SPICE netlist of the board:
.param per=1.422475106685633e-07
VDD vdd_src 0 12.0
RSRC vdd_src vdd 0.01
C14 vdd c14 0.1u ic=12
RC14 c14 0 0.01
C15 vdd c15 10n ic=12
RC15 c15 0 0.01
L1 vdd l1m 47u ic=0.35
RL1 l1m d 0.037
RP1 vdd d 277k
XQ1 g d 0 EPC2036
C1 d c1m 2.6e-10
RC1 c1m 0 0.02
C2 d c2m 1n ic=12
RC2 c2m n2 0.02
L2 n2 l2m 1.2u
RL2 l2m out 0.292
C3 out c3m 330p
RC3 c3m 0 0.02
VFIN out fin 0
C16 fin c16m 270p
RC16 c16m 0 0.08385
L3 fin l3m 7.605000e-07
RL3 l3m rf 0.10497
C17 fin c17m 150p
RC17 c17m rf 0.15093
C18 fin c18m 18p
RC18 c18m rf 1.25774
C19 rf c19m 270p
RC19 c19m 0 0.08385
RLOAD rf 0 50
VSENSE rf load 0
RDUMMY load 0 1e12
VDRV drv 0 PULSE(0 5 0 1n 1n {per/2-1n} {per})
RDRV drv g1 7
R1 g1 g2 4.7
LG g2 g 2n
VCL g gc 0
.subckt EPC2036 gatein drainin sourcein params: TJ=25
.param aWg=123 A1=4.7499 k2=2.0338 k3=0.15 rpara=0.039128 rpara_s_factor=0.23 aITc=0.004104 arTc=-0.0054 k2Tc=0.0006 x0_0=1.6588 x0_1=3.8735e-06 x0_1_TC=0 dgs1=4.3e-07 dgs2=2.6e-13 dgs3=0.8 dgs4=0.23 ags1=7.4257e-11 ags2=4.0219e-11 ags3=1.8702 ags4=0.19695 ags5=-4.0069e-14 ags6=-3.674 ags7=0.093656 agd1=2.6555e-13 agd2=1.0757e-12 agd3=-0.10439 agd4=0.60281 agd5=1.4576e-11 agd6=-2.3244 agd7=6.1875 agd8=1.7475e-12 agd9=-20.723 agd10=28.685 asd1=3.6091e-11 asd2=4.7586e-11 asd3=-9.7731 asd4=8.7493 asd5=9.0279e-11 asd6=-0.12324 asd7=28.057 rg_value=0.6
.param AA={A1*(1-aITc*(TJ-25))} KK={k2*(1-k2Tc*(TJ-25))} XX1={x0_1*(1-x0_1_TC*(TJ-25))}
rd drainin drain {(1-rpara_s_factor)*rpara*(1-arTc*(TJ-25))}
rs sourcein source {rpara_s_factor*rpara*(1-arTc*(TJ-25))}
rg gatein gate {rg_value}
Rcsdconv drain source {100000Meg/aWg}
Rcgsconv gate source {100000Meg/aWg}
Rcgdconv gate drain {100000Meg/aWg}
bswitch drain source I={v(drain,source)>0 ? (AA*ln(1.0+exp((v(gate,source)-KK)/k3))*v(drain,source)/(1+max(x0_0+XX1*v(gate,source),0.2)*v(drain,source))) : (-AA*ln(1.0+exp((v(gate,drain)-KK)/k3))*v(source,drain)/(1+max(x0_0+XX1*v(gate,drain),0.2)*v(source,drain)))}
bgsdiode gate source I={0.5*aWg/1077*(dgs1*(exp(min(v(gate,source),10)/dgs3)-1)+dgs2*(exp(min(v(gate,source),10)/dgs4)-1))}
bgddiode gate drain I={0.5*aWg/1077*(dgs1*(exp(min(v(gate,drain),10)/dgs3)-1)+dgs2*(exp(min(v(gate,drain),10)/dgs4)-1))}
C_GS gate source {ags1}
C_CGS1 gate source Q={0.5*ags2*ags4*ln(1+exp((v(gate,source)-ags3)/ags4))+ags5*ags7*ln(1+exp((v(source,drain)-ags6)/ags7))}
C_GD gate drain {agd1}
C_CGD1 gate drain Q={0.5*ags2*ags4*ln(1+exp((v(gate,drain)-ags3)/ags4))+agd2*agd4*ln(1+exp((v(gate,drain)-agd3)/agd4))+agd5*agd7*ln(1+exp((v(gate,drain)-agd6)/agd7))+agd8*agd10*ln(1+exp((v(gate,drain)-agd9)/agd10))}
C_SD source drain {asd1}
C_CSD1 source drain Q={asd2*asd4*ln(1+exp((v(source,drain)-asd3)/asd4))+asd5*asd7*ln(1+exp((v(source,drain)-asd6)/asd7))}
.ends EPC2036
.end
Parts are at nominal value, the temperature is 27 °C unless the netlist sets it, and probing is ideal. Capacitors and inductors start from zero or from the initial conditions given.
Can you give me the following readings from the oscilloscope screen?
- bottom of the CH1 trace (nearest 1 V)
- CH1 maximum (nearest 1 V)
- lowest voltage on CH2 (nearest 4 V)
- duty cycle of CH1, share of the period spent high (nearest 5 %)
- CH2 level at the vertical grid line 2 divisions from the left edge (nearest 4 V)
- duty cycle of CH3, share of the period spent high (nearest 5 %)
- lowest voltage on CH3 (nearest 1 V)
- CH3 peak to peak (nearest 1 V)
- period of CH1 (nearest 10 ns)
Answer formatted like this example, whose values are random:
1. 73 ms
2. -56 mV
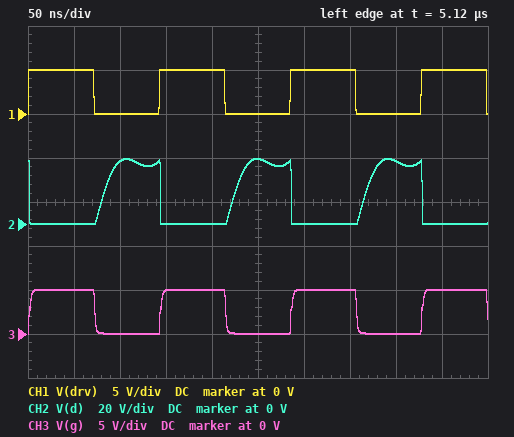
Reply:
1. 0 V
2. 5 V
3. 0 V
4. 50 %
5. 28 V
6. 50 %
7. 0 V
8. 5 V
9. 140 ns
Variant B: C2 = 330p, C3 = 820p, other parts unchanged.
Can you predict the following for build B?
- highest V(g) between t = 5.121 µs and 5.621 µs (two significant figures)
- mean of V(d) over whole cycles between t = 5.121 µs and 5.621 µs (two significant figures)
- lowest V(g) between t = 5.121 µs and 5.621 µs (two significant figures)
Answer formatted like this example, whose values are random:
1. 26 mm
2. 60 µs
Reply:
1. 5.0 V
2. 11 V
3. 10 mV
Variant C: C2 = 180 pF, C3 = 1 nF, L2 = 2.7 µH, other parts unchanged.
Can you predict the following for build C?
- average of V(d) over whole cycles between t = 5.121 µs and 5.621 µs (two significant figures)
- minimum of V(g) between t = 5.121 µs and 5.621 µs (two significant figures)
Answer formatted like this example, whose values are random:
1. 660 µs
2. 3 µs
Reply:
1. 11 V
2. 7.8 mV
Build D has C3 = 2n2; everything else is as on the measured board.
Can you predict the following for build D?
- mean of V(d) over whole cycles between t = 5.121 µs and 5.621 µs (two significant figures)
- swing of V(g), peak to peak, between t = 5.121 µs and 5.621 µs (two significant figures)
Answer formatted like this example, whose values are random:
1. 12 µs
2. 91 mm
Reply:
1. 13 V
2. 5.3 V
